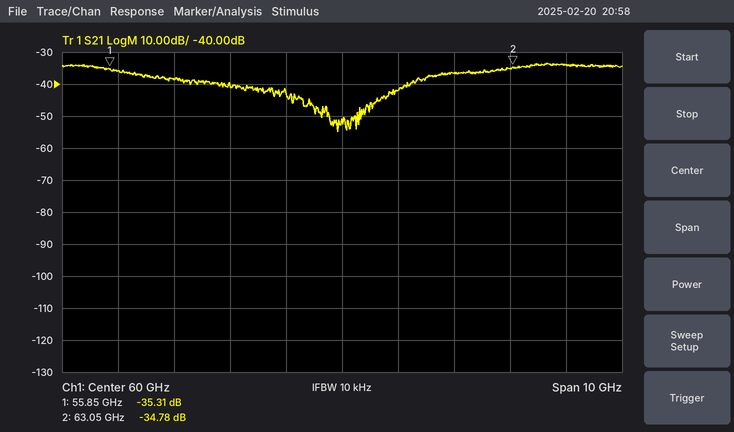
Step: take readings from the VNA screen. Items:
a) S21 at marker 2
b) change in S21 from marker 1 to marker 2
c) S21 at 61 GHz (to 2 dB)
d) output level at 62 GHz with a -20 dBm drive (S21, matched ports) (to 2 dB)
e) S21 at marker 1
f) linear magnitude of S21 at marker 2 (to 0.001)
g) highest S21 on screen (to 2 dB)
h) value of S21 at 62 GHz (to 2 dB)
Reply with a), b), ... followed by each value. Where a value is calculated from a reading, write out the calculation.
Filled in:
a) -34.78 dB
b) -34.78 − (-35.31) = 0.53 dB
c) -42 dB
d) -20 dBm + (-36 dB) = -56 dBm
e) -35.31 dB
f) 10^(-34.78/20) ≈ 0.018
g) -34 dB
h) -36 dB
